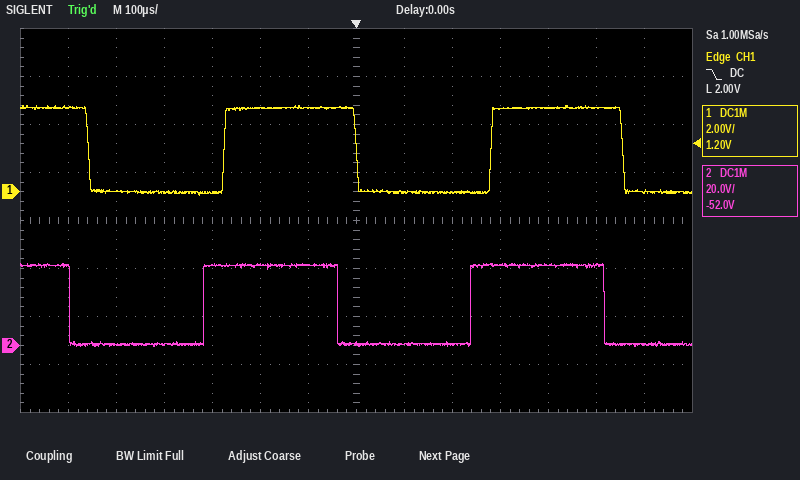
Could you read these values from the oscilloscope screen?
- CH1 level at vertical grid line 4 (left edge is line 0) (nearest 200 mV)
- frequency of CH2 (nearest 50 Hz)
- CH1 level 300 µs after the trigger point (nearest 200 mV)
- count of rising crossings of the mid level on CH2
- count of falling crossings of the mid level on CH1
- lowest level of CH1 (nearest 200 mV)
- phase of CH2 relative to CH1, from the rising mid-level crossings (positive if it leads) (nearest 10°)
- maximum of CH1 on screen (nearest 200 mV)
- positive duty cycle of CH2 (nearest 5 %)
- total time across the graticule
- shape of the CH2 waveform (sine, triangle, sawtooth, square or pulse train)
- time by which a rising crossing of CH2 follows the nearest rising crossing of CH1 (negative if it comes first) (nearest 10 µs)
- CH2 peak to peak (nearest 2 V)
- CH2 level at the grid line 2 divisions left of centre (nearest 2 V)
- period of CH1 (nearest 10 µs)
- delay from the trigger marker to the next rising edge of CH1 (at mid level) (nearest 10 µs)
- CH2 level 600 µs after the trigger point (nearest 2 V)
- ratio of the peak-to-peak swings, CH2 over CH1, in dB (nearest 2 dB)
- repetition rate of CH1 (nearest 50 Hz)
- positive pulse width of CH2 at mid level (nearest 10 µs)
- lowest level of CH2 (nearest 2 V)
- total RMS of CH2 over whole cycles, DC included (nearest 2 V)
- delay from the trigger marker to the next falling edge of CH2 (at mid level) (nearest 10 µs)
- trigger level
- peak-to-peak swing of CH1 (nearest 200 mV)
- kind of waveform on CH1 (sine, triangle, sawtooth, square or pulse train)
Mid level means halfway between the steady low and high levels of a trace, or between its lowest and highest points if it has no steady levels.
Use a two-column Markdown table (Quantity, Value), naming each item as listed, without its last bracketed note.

| Quantity | Value |
|---|---|
| CH1 level at vertical grid line 4 (left edge is line 0) | 0.0 V |
| frequency of CH2 | 1.80 kHz |
| CH1 level 300 µs after the trigger point | 3.4 V |
| count of rising crossings of the mid level on CH2 | 2 |
| count of falling crossings of the mid level on CH1 | 3 |
| lowest level of CH1 | -200 mV |
| phase of CH2 relative to CH1, from the rising mid-level crossings (positive if it leads) | +30° |
| maximum of CH1 on screen | 3.6 V |
| positive duty cycle of CH2 | 50 % |
| total time across the graticule | 1.4 ms |
| shape of the CH2 waveform | square |
| time by which a rising crossing of CH2 follows the nearest rising crossing of CH1 (negative if it comes first) | -40 µs |
| CH2 peak to peak | 34 V |
| CH2 level at the grid line 2 divisions left of centre | 34 V |
| period of CH1 | 560 µs |
| delay from the trigger marker to the next rising edge of CH1 (at mid level) | 280 µs |
| CH2 level 600 µs after the trigger point | 0 V |
| ratio of the peak-to-peak swings, CH2 over CH1, in dB | 20 dB |
| repetition rate of CH1 | 1.80 kHz |
| positive pulse width of CH2 at mid level | 280 µs |
| lowest level of CH2 | 0 V |
| total RMS of CH2 over whole cycles, DC included | 24 V |
| delay from the trigger marker to the next falling edge of CH2 (at mid level) | 520 µs |
| trigger level | 2.00 V |
| peak-to-peak swing of CH1 | 3.8 V |
| kind of waveform on CH1 | square |
